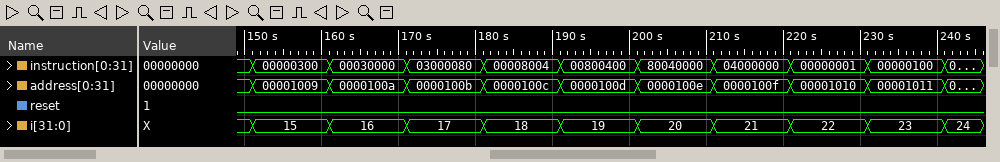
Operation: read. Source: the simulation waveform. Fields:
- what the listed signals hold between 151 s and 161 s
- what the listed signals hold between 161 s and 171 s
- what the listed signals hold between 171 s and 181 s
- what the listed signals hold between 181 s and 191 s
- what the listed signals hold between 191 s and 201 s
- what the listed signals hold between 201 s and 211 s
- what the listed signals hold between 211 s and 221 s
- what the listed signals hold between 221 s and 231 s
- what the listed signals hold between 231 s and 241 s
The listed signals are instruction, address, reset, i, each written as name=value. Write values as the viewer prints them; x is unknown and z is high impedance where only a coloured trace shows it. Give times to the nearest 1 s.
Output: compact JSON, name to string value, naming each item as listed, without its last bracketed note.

{"what the listed signals hold between 151 s and 161 s": "instruction=00000300, address=00001009, reset=0, i=15", "what the listed signals hold between 161 s and 171 s": "instruction=00030000, address=0000100a, reset=0, i=16", "what the listed signals hold between 171 s and 181 s": "instruction=03000080, address=0000100b, reset=0, i=17", "what the listed signals hold between 181 s and 191 s": "instruction=00008004, address=0000100c, reset=0, i=18", "what the listed signals hold between 191 s and 201 s": "instruction=00800400, address=0000100d, reset=0, i=19", "what the listed signals hold between 201 s and 211 s": "instruction=80040000, address=0000100e, reset=0, i=20", "what the listed signals hold between 211 s and 221 s": "instruction=04000000, address=0000100f, reset=0, i=21", "what the listed signals hold between 221 s and 231 s": "instruction=00000001, address=00001010, reset=0, i=22", "what the listed signals hold between 231 s and 241 s": "instruction=00000100, address=00001011, reset=0, i=23"}
